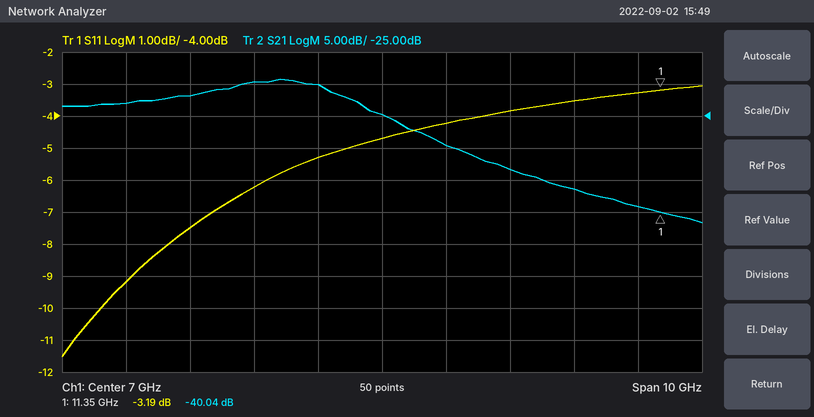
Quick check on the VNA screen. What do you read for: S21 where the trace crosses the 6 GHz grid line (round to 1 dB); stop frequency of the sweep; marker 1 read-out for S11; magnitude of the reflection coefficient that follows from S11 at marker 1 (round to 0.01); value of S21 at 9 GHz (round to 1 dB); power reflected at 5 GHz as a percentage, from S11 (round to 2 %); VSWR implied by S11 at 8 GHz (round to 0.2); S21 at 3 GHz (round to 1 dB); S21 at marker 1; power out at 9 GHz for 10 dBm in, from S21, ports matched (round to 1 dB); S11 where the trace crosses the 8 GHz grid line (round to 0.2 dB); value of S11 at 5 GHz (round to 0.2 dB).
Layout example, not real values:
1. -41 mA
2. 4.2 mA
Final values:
1. -20 dB
2. 12 GHz
3. -3.19 dB
4. 0.69
5. -33 dB
6. 24 %
7. 4.2
8. -23 dB
9. -40.04 dB
10. -23 dBm
11. -4.2 dB
12. -6.2 dB
